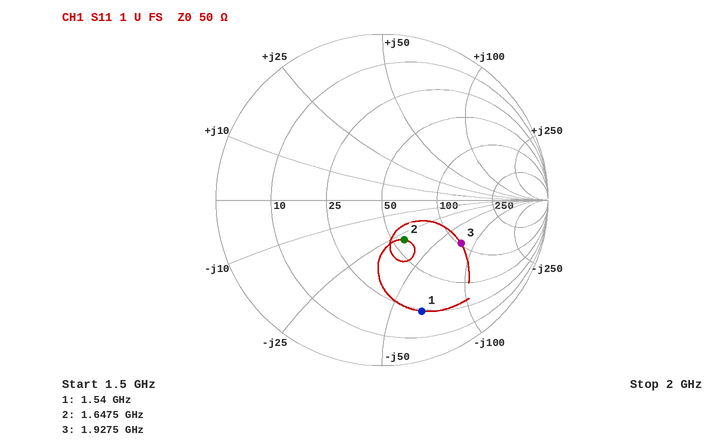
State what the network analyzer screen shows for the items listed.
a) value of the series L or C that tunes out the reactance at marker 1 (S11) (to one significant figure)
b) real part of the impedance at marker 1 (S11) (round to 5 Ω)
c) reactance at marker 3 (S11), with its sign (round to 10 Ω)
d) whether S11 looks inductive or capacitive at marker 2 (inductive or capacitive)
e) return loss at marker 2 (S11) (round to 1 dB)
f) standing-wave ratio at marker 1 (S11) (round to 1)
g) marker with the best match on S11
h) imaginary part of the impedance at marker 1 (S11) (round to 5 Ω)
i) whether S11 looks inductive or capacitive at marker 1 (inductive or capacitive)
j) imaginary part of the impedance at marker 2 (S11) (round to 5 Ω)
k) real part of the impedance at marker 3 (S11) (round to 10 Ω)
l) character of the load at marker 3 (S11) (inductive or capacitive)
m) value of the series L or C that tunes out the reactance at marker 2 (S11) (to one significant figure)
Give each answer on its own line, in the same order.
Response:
7 nH
25 Ω
-80 Ω
capacitive
11 dB
6
marker 2
-65 Ω
capacitive
-30 Ω
100 Ω
capacitive
3 nH
